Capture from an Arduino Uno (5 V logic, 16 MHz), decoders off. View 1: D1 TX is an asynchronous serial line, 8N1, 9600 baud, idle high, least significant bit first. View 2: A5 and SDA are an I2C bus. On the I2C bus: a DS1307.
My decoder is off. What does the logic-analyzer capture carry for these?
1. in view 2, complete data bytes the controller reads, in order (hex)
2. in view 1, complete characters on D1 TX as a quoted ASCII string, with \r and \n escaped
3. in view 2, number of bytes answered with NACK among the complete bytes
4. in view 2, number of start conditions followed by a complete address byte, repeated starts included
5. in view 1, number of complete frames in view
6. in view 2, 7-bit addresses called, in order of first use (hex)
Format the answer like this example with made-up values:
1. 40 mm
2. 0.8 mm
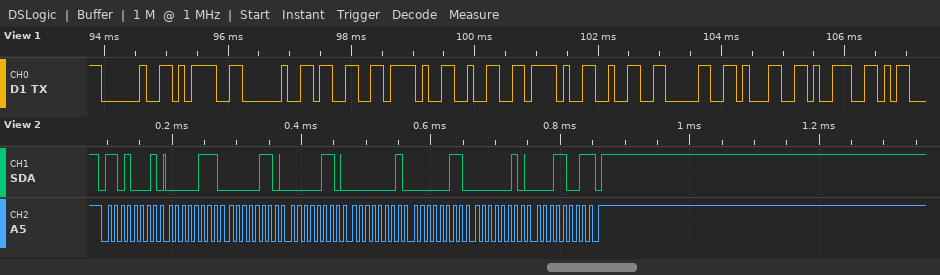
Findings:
1. 07 06 06 01 03 02 19
2. " = 3/2/2019"
3. 1
4. 1
5. 11
6. 0x68
